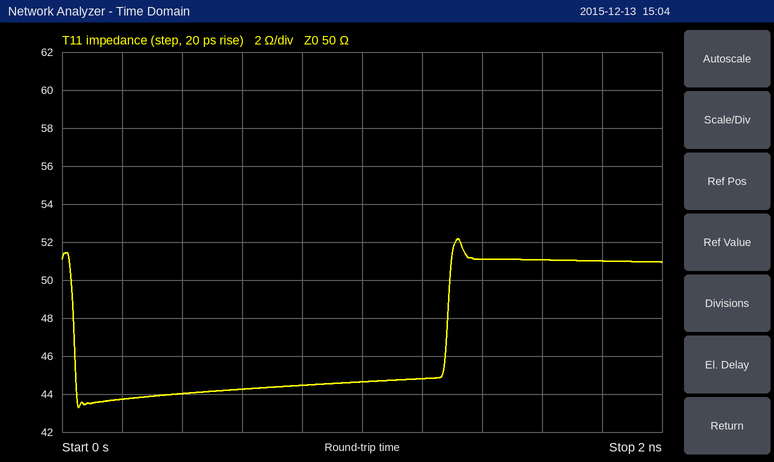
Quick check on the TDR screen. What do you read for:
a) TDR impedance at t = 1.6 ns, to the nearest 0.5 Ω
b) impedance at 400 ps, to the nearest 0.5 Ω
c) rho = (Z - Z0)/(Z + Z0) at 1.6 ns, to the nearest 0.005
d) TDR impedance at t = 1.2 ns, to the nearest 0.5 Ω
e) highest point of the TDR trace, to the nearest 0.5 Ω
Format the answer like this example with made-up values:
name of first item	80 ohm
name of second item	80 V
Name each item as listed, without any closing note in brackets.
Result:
TDR impedance at t = 1.6 ns, to the nearest 0.5 Ω	51.0 Ω
impedance at 400 ps, to the nearest 0.5 Ω	44.0 Ω
rho = (Z - Z0)/(Z + Z0) at 1.6 ns, to the nearest 0.005	+0.010
TDR impedance at t = 1.2 ns, to the nearest 0.5 Ω	45.0 Ω
highest point of the TDR trace, to the nearest 0.5 Ω	52.0 Ω
